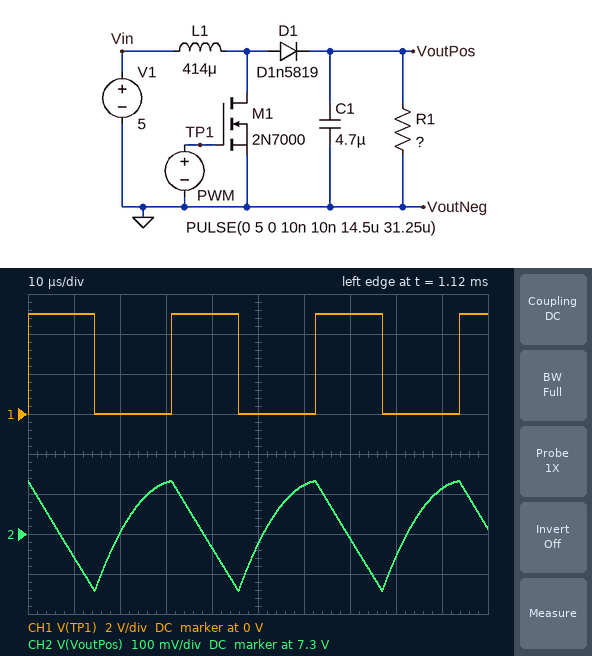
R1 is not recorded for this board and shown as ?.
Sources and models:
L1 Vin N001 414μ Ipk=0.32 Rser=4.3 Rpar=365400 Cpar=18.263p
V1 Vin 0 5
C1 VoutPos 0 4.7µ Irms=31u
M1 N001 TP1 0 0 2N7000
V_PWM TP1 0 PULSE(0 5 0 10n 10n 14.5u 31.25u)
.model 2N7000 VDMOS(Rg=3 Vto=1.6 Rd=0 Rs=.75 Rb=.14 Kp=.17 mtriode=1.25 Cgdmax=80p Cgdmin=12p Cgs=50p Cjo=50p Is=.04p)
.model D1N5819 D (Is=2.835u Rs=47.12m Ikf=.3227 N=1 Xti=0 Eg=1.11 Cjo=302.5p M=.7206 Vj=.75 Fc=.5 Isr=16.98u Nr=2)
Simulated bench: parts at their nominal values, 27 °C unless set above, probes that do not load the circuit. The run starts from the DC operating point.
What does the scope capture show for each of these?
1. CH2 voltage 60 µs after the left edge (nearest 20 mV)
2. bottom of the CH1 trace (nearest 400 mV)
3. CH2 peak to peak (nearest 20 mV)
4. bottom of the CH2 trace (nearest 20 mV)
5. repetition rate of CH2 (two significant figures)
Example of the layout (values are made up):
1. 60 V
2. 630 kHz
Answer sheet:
1. 7.42 V
2. 0 V
3. 280 mV
4. 7.16 V
5. 32 kHz
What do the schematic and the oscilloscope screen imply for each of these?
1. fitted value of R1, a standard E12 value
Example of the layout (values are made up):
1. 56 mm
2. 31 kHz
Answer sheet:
1. 82 Ω
